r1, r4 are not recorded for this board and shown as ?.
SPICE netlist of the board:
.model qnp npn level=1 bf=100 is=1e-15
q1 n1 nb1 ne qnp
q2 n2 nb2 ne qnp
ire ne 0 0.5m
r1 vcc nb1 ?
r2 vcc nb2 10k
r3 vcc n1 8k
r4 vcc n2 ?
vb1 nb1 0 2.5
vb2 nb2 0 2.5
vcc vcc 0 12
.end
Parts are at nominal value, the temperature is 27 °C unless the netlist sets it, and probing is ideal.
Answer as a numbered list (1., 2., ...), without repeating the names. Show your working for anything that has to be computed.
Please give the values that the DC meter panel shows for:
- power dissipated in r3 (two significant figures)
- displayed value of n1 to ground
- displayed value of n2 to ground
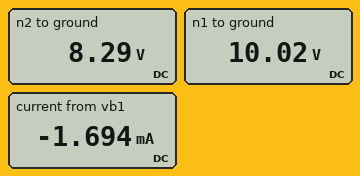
1. (12 V - 10.02 V)^2 / 8 kΩ = 490 µW
2. 10.02 V
3. 8.29 V
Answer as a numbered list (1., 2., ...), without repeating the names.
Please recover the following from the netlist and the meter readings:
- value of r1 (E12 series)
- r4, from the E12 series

1. 5.6 kΩ
2. 15 kΩ
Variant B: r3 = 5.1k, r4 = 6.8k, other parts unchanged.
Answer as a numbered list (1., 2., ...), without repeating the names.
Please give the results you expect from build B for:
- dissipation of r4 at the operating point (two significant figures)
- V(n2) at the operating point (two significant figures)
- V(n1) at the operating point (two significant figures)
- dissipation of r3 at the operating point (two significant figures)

1. 420 µW
2. 10 V
3. 11 V
4. 310 µW
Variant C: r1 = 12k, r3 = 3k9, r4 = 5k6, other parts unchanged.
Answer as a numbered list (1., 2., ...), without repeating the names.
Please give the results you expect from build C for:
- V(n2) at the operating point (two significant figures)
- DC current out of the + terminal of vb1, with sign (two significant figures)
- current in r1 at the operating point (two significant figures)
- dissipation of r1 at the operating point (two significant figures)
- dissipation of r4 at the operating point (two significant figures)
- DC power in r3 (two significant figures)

1. 11 V
2. -790 µA
3. 790 µA
4. 7.5 mW
5. 340 µW
6. 240 µW
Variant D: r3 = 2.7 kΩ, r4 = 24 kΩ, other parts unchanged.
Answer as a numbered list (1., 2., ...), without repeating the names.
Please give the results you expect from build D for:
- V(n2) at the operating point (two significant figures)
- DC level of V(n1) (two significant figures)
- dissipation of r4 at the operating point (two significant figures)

1. 6.1 V
2. 11 V
3. 1.5 mW
